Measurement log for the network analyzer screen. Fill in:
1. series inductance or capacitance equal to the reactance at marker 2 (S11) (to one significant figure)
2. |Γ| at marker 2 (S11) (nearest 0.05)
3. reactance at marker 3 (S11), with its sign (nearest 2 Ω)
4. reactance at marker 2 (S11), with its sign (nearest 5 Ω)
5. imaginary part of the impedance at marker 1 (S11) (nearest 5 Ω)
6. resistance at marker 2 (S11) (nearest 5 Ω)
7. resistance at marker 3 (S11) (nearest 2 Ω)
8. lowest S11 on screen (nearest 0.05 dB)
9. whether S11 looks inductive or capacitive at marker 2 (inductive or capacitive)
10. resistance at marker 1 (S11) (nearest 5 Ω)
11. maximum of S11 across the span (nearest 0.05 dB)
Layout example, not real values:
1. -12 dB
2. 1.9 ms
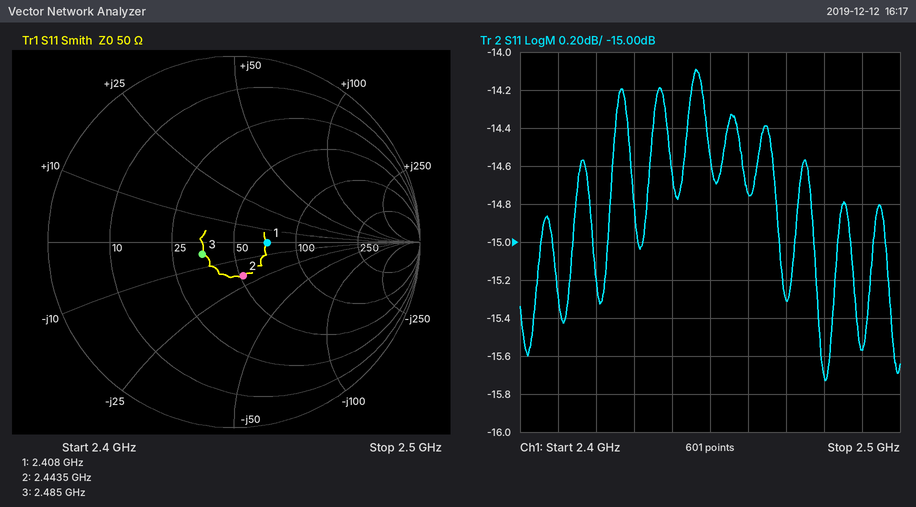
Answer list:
1. 3 pF
2. 0.20
3. -4 Ω
4. -20 Ω
5. 0 Ω
6. 50 Ω
7. 36 Ω
8. -15.75 dB
9. capacitive
10. 70 Ω
11. -14.10 dB
